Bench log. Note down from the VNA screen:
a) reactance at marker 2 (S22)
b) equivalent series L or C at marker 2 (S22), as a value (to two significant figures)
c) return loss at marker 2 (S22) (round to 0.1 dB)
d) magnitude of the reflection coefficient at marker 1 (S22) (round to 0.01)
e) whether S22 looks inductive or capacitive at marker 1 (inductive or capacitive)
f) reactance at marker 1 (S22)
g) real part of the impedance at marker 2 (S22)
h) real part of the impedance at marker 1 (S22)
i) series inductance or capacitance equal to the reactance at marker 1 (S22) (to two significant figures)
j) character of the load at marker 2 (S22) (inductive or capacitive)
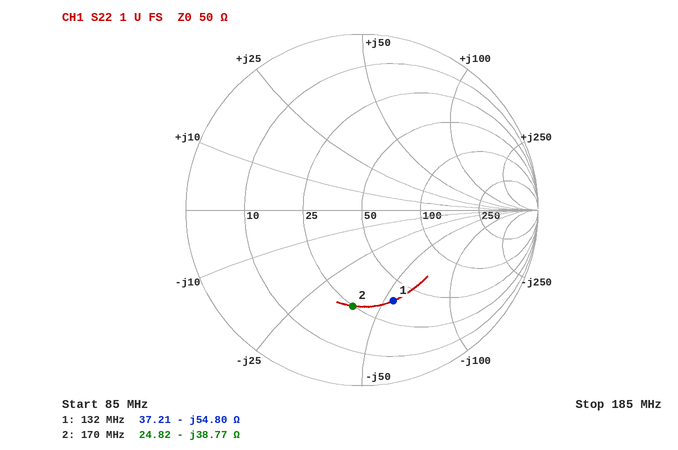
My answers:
-38.77 Ω
24 pF
5.2 dB
0.55
capacitive
-54.80 Ω
24.82 Ω
37.21 Ω
22 pF
capacitive
